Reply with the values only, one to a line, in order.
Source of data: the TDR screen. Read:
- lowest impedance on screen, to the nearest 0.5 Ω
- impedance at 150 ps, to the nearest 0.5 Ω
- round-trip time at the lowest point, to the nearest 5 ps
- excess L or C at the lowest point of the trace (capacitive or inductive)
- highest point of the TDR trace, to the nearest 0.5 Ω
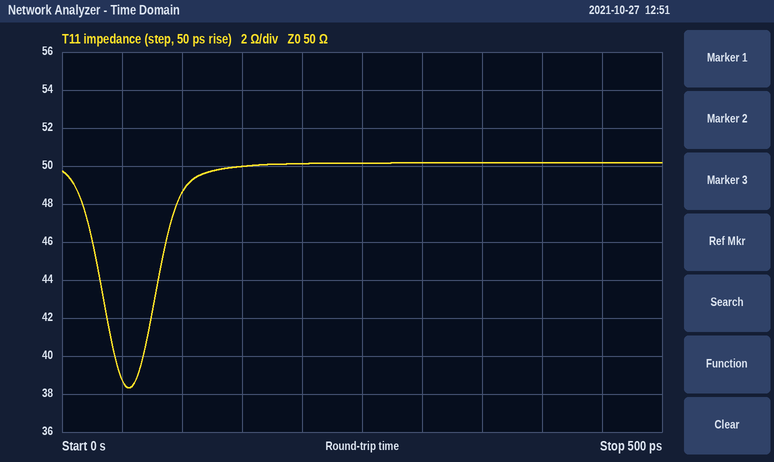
38.5 Ω
50.0 Ω
55 ps
capacitive
50.0 Ω
